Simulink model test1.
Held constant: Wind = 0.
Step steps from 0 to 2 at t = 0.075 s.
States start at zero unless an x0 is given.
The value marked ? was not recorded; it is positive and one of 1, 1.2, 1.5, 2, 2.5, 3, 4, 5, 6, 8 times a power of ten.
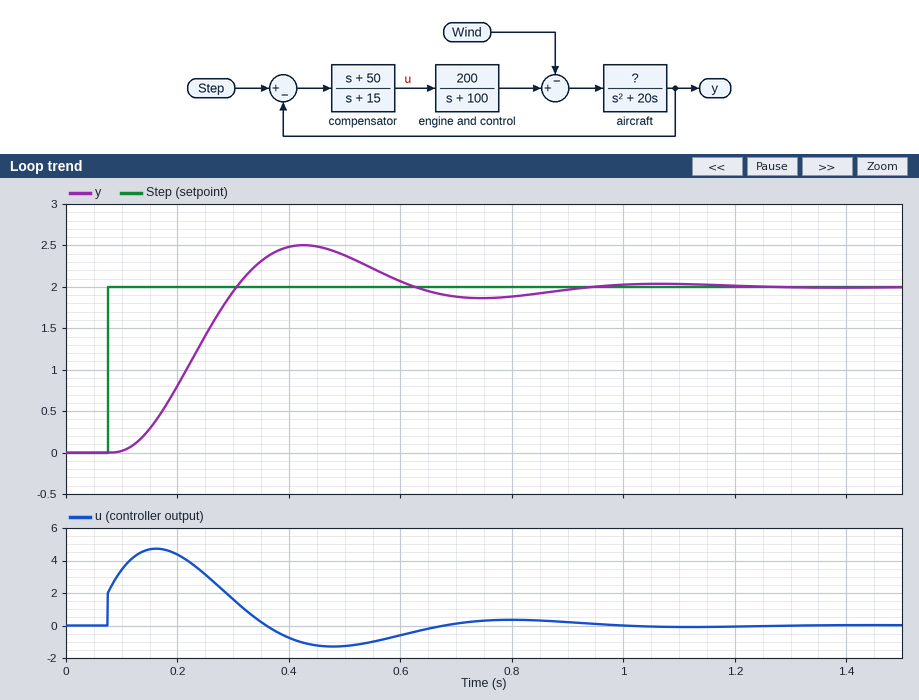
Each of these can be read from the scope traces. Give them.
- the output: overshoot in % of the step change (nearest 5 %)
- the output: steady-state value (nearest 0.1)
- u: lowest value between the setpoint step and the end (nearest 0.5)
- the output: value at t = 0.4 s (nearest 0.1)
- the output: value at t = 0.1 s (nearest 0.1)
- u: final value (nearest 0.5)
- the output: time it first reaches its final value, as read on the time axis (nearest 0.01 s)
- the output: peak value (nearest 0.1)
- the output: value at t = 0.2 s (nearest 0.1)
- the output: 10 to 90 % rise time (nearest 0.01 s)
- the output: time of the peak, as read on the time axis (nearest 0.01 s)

25 %
2.0
-1.5
2.5
0.0
0.0
0.31 s
2.5
0.8
0.15 s
0.43 s
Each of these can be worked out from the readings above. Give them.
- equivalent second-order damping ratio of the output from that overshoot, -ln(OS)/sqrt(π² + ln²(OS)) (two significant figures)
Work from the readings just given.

0.40
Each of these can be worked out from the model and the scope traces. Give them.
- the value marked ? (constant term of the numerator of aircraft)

30
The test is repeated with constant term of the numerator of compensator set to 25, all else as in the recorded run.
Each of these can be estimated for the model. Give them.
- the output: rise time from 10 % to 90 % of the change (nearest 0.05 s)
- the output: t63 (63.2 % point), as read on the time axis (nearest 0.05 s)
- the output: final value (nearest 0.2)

0.30 s
0.30 s
2.0
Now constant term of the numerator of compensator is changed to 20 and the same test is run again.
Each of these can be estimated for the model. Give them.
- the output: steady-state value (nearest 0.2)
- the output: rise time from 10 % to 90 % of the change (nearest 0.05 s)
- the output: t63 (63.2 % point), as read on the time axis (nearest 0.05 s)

2.0
0.40 s
0.35 s
